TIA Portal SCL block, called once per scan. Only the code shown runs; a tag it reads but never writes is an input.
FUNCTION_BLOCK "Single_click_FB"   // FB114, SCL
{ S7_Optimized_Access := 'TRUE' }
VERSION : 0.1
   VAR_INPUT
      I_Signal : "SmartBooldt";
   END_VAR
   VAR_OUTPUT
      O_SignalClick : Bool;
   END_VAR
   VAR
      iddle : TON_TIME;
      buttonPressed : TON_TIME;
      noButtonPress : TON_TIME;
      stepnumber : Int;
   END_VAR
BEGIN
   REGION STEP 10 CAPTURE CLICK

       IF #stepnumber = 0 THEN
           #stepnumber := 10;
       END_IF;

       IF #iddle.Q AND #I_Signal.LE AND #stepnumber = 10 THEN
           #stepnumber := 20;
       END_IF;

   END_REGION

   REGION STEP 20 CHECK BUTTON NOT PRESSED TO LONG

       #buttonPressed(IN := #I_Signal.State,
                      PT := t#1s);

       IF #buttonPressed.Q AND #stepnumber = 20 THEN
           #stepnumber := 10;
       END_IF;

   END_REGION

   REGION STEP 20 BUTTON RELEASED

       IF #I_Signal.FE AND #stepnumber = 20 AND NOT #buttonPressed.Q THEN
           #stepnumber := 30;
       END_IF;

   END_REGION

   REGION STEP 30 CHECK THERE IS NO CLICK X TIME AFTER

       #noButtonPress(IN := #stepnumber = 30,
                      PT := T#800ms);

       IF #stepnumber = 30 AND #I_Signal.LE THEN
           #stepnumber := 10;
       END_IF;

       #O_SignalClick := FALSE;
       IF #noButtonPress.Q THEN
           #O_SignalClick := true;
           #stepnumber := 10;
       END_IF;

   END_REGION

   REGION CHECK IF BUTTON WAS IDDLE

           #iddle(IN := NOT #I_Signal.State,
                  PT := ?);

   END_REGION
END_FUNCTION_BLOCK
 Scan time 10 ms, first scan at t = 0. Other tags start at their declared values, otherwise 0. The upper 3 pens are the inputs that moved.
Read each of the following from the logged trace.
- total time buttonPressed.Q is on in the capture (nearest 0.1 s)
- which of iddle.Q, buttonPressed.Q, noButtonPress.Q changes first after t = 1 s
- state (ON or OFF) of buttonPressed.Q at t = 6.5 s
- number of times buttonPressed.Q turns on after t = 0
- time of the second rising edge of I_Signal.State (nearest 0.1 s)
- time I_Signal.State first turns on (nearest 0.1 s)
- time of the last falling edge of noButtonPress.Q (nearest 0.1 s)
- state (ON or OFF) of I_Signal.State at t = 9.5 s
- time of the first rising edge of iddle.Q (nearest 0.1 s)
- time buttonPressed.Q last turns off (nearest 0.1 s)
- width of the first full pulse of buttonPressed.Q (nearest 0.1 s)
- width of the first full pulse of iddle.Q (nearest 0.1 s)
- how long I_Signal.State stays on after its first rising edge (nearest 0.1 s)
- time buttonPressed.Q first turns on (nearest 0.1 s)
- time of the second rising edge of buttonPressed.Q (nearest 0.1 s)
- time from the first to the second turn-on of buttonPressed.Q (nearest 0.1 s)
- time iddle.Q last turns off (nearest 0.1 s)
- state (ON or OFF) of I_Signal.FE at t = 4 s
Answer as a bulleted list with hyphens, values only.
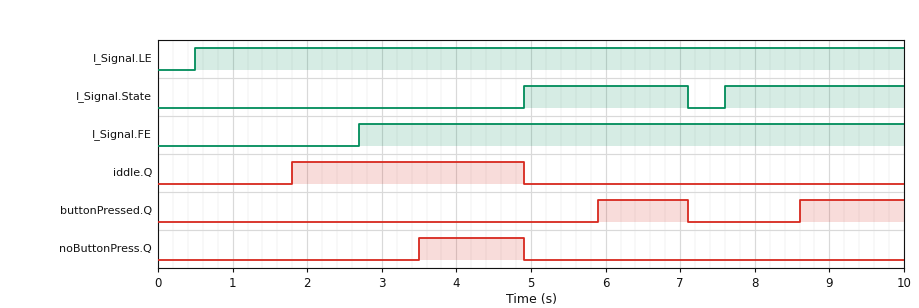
- 2.6 s
- iddle.Q
- ON
- 2
- 7.6 s
- 4.9 s
- 4.9 s
- ON
- 1.8 s
- 7.1 s
- 1.2 s
- 3.1 s
- 2.2 s
- 5.9 s
- 8.6 s
- 2.7 s
- 4.9 s
- ON
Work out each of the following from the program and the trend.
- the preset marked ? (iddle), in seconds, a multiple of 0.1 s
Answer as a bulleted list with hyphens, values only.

- 1.8 s
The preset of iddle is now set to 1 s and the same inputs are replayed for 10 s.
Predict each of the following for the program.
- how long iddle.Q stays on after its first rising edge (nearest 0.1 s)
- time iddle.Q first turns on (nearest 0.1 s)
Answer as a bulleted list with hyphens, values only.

- 3.9 s
- 1.0 s
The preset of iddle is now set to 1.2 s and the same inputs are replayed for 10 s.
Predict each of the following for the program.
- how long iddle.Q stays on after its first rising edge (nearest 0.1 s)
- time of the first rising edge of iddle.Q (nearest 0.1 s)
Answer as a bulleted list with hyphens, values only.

- 3.7 s
- 1.2 s
